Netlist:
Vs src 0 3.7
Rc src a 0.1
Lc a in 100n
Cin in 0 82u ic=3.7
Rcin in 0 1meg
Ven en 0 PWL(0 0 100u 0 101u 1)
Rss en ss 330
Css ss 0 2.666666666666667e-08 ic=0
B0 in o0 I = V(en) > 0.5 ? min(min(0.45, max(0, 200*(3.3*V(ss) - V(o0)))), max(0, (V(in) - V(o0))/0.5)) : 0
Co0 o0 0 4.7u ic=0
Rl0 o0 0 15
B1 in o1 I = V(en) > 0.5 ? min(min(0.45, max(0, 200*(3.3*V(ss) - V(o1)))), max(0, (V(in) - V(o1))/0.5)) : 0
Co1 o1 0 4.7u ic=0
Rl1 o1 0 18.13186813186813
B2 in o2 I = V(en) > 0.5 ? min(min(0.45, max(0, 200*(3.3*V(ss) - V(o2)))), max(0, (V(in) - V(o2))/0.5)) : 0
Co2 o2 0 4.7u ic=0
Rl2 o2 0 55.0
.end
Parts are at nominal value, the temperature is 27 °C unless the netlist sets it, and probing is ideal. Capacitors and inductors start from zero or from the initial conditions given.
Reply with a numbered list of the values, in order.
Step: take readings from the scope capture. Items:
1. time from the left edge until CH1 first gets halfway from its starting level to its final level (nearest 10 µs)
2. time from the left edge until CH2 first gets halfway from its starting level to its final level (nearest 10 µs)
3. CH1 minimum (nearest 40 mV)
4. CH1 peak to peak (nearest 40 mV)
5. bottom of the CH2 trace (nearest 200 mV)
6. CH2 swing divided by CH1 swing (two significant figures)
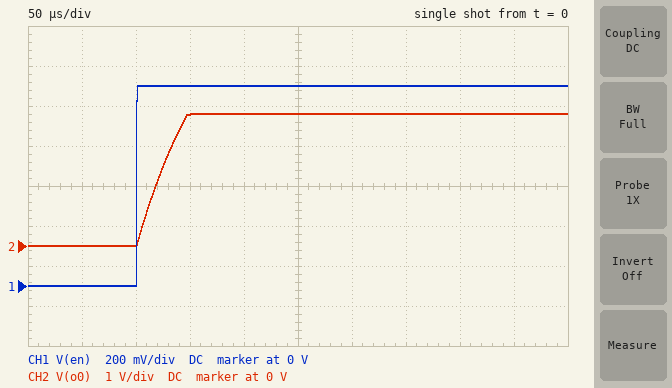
1. 100 µs
2. 120 µs
3. 0 V
4. 1.00 V
5. 0 V
6. 3.3
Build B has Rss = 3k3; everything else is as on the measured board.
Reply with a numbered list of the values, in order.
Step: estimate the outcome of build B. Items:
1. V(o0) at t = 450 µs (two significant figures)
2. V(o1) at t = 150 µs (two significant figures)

1. 3.2 V
2. 1.4 V
